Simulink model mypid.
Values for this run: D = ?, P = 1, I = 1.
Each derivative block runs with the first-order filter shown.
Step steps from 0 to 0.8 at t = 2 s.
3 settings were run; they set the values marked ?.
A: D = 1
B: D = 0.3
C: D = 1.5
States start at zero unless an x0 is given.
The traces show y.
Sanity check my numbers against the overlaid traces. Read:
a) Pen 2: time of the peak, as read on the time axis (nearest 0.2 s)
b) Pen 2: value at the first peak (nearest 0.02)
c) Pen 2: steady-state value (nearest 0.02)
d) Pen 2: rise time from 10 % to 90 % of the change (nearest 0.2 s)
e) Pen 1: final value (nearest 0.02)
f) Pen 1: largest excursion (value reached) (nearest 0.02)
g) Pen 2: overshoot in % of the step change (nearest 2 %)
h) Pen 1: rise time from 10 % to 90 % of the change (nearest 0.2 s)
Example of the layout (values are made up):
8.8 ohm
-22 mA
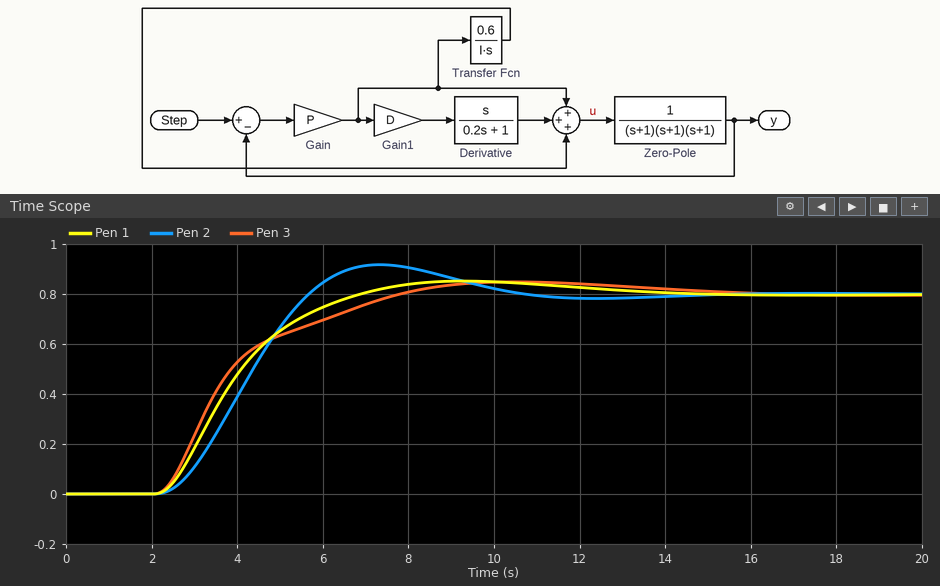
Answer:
7.4 s
0.92
0.80
2.4 s
0.80
0.86
14 %
3.0 s
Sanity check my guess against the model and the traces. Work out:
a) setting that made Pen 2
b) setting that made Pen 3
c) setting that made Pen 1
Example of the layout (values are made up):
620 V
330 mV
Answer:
B
C
A
